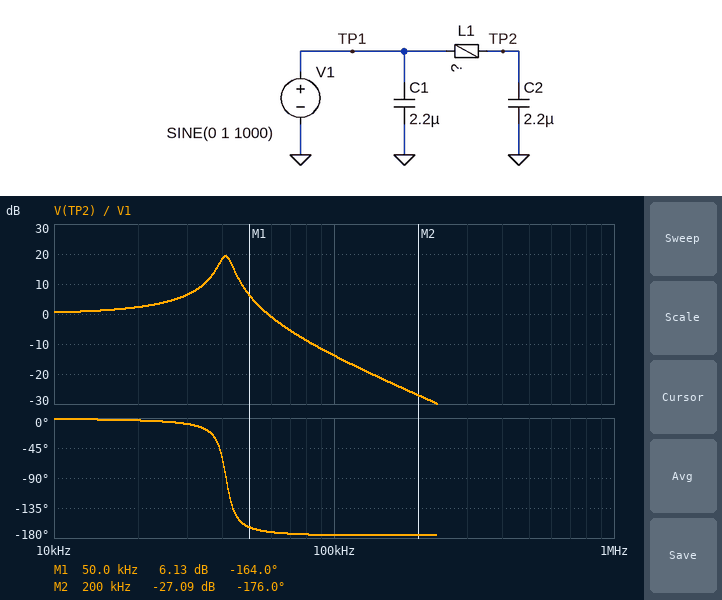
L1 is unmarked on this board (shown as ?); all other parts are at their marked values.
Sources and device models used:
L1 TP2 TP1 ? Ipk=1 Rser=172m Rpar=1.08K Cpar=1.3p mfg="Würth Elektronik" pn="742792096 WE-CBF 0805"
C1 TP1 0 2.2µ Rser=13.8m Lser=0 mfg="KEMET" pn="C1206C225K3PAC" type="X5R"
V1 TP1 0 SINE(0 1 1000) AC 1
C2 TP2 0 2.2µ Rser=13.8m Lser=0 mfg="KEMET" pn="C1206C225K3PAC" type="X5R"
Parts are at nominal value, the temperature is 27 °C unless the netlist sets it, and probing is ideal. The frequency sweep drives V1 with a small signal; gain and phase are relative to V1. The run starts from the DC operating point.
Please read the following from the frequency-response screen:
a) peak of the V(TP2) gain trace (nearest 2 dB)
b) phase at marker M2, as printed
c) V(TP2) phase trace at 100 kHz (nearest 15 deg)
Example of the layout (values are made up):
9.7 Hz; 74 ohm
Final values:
20 dB; -176.0 deg; -180 deg
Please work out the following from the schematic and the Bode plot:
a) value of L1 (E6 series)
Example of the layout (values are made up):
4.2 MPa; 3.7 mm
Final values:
6.8 µH
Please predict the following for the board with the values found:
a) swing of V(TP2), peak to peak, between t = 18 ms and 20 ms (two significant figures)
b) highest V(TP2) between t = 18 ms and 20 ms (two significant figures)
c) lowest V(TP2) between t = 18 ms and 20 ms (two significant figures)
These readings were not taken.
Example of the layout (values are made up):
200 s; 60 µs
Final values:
2.0 V; 1.0 V; -1.0 V
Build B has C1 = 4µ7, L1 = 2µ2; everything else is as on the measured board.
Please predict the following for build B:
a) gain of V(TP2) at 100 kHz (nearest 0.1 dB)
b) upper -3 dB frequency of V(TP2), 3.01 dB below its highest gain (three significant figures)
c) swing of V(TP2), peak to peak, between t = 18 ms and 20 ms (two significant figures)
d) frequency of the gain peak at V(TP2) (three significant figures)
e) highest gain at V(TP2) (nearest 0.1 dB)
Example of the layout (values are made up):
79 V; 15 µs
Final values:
0.5 dB; 78.2 kHz; 2.0 V; 71.7 kHz; 14.6 dB
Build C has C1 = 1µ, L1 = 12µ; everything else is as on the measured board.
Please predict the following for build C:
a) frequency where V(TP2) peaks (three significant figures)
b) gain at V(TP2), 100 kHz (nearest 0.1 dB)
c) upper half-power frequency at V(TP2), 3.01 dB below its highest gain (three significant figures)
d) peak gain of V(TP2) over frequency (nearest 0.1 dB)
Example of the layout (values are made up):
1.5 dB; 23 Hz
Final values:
30.9 kHz; -19.5 dB; 32.2 kHz; 21.8 dB
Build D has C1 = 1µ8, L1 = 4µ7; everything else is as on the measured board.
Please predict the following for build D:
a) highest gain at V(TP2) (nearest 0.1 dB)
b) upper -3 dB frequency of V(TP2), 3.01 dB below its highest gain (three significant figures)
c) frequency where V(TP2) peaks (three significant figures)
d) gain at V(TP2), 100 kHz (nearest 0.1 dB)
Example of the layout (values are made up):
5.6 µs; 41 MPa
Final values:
17.8 dB; 52.4 kHz; 49.3 kHz; -9.8 dB
